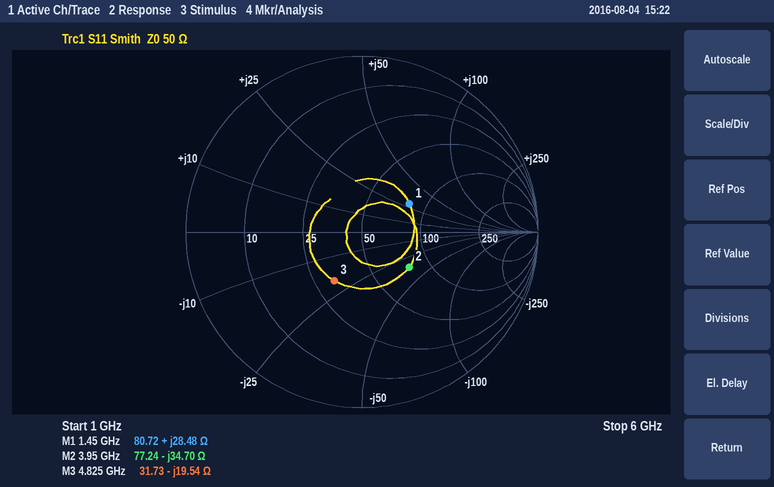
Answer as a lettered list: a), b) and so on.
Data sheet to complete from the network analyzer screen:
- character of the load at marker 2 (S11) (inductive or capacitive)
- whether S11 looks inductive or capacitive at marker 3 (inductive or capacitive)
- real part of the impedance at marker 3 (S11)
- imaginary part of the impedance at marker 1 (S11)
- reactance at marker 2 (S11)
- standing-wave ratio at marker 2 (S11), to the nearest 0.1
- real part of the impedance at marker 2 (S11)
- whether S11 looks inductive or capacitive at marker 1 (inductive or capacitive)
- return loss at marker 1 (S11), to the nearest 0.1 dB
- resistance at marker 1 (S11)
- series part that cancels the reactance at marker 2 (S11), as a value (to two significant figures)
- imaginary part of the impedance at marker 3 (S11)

a) capacitive
b) capacitive
c) 31.73 Ω
d) +28.48 Ω
e) -34.70 Ω
f) 2.0
g) 77.24 Ω
h) inductive
i) 10.1 dB
j) 80.72 Ω
k) 1.4 nH
l) -19.54 Ω
